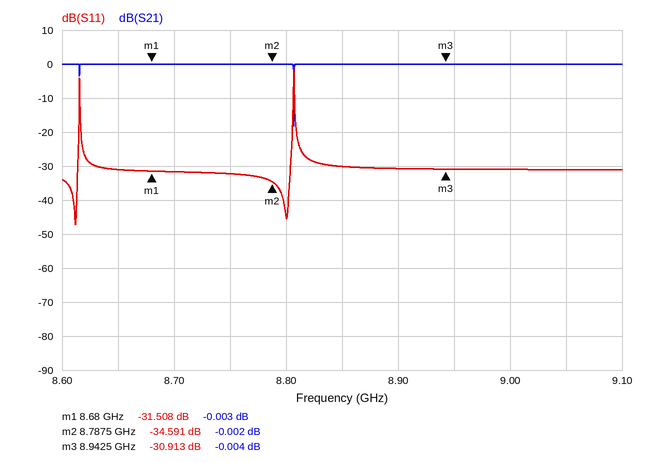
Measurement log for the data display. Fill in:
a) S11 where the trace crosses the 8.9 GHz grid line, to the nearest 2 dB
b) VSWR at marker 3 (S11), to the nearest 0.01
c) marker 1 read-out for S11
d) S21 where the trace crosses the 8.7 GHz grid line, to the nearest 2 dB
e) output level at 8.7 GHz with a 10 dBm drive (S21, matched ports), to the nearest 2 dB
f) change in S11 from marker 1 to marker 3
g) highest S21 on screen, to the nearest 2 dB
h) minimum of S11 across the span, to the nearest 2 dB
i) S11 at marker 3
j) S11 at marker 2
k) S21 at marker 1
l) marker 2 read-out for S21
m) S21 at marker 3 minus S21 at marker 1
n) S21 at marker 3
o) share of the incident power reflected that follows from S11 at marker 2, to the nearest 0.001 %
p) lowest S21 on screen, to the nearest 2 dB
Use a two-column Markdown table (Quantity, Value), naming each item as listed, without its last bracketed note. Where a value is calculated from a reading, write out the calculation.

| Quantity | Value |
|---|---|
| S11 where the trace crosses the 8.9 GHz grid line, to the nearest 2 dB | -30 dB |
| VSWR at marker 3 (S11), to the nearest 0.01 | (1 + 0.0285)/(1 − 0.0285) ≈ 1.06 |
| marker 1 read-out for S11 | -31.508 dB |
| S21 where the trace crosses the 8.7 GHz grid line, to the nearest 2 dB | 0 dB |
| output level at 8.7 GHz with a 10 dBm drive (S21, matched ports), to the nearest 2 dB | 10 dBm + (0 dB) = 10 dBm |
| change in S11 from marker 1 to marker 3 | -30.913 − (-31.508) = 0.595 dB |
| highest S21 on screen, to the nearest 2 dB | 0 dB |
| minimum of S11 across the span, to the nearest 2 dB | -48 dB |
| S11 at marker 3 | -30.913 dB |
| S11 at marker 2 | -34.591 dB |
| S21 at marker 1 | -0.003 dB |
| marker 2 read-out for S21 | -0.002 dB |
| S21 at marker 3 minus S21 at marker 1 | -0.004 − (-0.003) = -0.001 dB |
| S21 at marker 3 | -0.004 dB |
| share of the incident power reflected that follows from S11 at marker 2, to the nearest 0.001 % | 10^(-34.591/10) ≈ 0.035 % |
| lowest S21 on screen, to the nearest 2 dB | -18 dB |
